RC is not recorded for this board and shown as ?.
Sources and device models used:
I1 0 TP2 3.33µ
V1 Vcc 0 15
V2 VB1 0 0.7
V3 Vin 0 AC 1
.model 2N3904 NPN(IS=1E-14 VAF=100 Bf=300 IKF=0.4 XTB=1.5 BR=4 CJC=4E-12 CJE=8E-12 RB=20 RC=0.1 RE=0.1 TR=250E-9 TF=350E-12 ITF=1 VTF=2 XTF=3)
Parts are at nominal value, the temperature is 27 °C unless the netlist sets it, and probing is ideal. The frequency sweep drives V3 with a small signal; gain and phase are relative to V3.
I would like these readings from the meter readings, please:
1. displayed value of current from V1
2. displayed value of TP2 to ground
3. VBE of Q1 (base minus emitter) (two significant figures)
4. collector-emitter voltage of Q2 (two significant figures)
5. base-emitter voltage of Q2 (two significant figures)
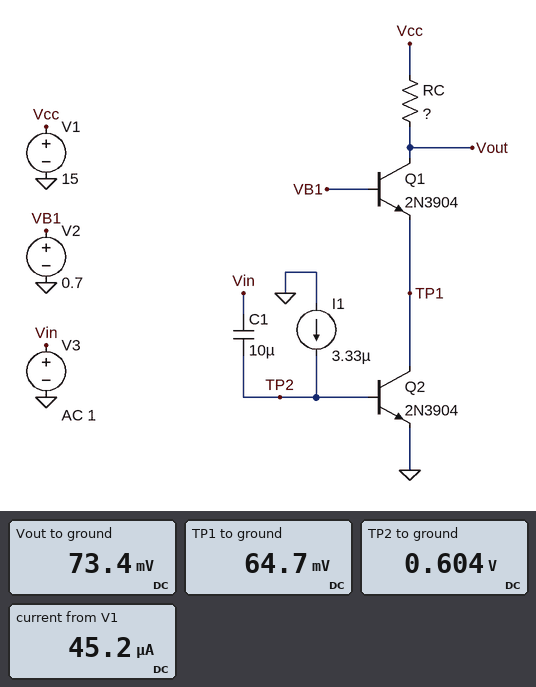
45.2 µA
0.604 V
640 mV
65 mV
600 mV
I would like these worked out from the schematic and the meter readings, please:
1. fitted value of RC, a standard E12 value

330 kΩ
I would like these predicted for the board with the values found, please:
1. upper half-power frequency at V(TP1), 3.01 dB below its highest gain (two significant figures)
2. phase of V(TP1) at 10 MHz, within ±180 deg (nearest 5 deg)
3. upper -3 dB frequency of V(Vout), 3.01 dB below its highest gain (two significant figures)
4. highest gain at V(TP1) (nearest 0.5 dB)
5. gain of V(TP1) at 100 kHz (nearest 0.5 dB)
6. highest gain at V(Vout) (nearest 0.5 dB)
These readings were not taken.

190 kHz
80 deg
180 kHz
2.0 dB
1.0 dB
3.0 dB
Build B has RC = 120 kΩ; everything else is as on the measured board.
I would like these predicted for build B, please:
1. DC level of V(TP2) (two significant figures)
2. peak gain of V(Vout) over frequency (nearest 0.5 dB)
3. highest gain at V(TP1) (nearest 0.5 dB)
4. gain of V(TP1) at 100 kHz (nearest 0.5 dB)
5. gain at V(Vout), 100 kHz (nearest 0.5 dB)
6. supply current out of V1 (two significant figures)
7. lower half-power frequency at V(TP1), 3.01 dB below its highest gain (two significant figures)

610 mV
10.5 dB
6.5 dB
5.5 dB
9.5 dB
120 µA
5.6 Hz
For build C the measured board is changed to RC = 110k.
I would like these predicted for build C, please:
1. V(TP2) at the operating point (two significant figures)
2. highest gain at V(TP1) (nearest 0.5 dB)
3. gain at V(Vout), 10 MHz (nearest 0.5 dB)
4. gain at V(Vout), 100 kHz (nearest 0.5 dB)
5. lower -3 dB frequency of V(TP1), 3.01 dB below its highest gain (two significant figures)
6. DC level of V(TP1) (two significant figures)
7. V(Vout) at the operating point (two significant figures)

610 mV
7.0 dB
-17.0 dB
10.5 dB
5.8 Hz
74 mV
94 mV
